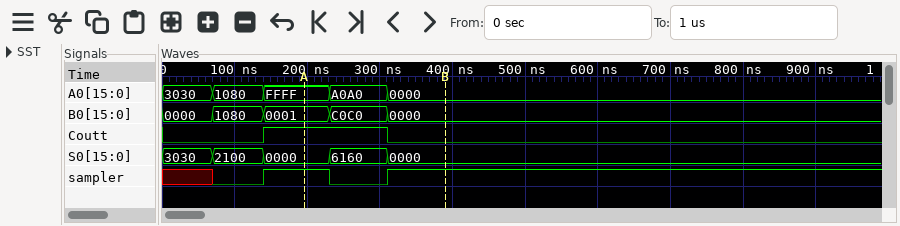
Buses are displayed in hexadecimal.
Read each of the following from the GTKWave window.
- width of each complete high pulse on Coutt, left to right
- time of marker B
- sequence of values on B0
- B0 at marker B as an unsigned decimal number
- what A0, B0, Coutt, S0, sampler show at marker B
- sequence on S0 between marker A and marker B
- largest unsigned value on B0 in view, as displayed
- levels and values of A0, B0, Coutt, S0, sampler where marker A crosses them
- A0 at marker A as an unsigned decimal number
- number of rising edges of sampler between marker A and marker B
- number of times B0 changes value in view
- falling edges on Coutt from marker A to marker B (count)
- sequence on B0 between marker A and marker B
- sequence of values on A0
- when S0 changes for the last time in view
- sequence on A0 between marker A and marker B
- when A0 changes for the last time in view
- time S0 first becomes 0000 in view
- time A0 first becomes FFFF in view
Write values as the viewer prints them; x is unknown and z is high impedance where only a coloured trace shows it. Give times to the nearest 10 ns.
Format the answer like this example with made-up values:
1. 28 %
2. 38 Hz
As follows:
1. 170 ns
2. 390 ns
3. 0000, 1080, 0001, C0C0, 0000
4. 0
5. A0=0000, B0=0000, Coutt=0, S0=0000, sampler=1
6. 0000, 6160, 0000
7. C0C0
8. A0=FFFF, B0=0001, Coutt=1, S0=0000, sampler=1
9. 65535
10. 1
11. 4
12. 1
13. 0001, C0C0, 0000
14. 3030, 1080, FFFF, A0A0, 0000
15. 310 ns
16. FFFF, A0A0, 0000
17. 310 ns
18. 140 ns
19. 140 ns
